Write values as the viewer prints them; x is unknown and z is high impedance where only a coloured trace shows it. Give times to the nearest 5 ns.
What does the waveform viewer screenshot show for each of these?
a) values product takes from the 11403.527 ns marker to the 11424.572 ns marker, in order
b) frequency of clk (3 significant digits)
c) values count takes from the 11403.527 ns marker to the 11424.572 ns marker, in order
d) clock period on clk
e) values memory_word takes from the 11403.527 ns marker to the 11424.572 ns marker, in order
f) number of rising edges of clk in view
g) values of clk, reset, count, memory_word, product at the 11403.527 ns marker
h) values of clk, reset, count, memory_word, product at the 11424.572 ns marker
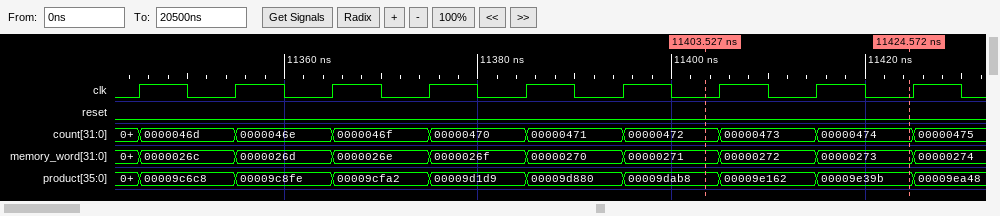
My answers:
00009dab8, 00009e162, 00009e39b
100 MHz
00000472, 00000473, 00000474
10 ns
00000271, 00000272, 00000273
9
clk=0, reset=0, count=00000472, memory_word=00000271, product=00009dab8
clk=0, reset=0, count=00000474, memory_word=00000273, product=00009e39b
